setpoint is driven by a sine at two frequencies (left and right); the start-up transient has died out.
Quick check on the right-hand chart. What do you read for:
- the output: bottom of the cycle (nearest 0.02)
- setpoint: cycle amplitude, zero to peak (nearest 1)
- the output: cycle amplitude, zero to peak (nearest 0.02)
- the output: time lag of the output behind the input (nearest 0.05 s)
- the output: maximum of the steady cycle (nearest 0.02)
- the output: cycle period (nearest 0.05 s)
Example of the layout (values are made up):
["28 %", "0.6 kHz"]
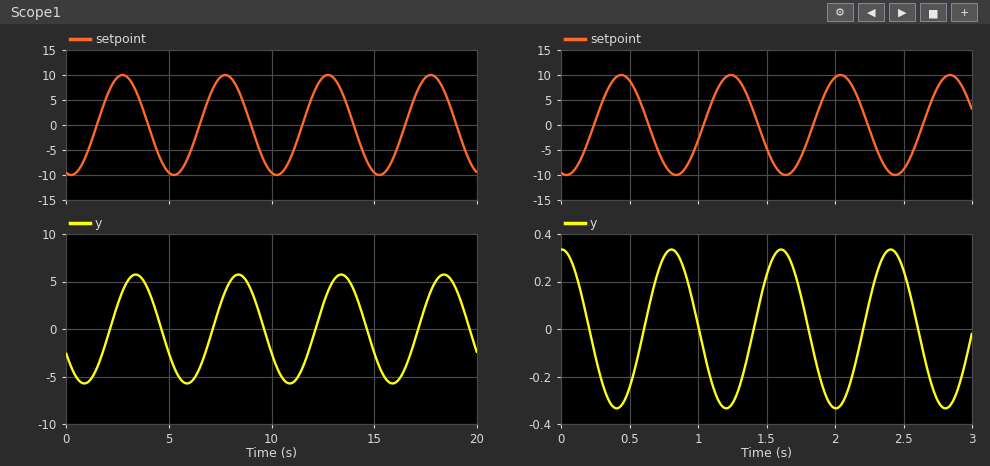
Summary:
["-0.34", "10", "0.34", "0.35 s", "0.34", "0.80 s"]
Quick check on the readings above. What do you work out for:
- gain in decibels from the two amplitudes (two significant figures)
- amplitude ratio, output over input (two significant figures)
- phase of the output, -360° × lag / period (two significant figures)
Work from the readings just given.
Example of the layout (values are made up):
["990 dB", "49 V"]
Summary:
["-29 dB", "0.034", "-160°"]
